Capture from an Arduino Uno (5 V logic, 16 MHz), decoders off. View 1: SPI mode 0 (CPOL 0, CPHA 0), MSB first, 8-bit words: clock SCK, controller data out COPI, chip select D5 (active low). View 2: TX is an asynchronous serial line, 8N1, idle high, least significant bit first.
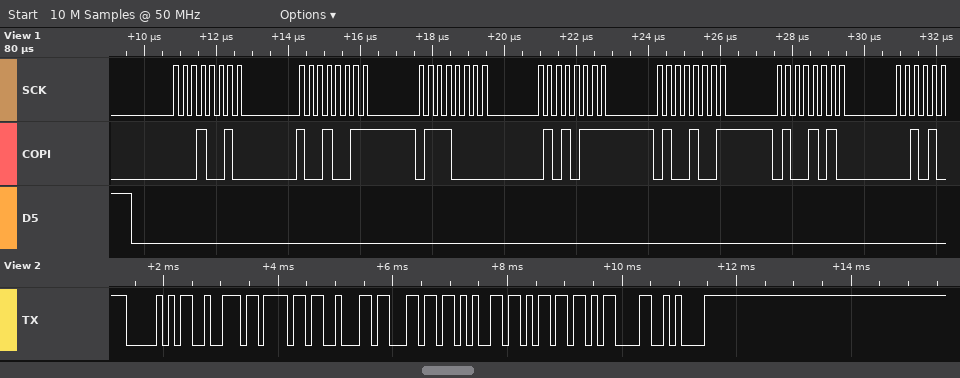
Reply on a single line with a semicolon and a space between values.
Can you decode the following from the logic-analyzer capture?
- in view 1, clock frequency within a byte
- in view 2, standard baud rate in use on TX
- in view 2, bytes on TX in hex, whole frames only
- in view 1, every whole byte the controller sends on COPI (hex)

4 MHz; 9600 baud; 0x50 0x72 0x6F 0x62 0x6C 0x65 0x6D 0x0D 0x0A; 12 93 70 57 49 4A
